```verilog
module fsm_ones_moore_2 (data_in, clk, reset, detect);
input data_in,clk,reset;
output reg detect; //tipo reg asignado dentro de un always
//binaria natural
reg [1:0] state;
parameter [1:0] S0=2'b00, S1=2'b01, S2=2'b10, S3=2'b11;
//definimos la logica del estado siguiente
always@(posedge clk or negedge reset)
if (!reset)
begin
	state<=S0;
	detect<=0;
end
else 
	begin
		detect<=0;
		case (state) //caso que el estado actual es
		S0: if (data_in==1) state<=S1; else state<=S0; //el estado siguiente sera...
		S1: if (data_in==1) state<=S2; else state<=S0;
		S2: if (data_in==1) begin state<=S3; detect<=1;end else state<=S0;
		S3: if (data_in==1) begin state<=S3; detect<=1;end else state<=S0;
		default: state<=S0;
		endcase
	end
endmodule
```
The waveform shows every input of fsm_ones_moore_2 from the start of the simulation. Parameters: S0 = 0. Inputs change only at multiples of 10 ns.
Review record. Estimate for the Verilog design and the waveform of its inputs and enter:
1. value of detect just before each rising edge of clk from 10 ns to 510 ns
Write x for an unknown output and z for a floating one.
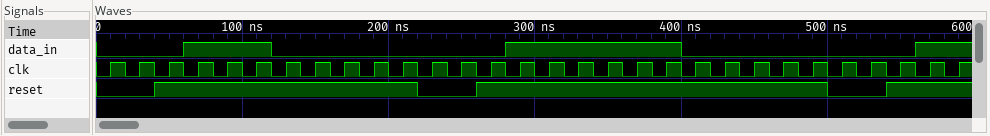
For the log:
0 0 0 0 0 0 1 0 0 0 0 0 0 0 0 0 0 1 1 1 1 0 0 0 0 0
